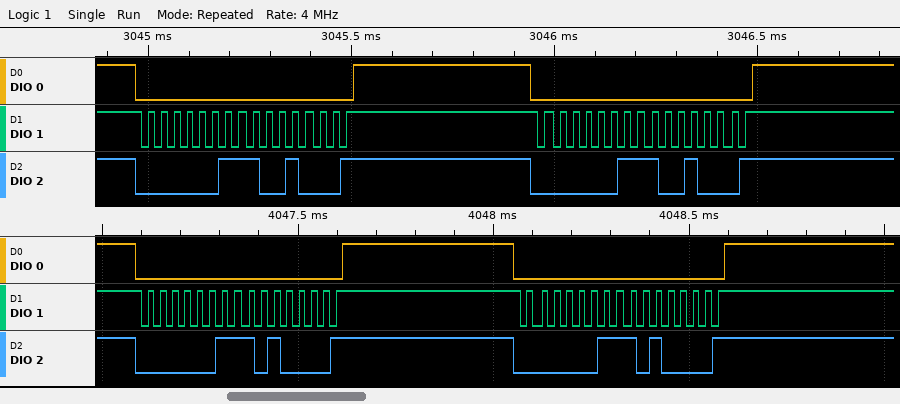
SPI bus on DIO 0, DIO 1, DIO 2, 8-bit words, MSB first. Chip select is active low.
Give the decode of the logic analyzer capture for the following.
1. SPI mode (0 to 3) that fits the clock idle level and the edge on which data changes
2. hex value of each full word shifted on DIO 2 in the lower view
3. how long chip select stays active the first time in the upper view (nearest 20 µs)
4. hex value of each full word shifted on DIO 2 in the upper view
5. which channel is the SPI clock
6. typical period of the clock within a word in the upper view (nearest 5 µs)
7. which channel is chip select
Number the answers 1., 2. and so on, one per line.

1. 3
2. 03, A1, 03, A1
3. 540 µs
4. 03, 91, 03, 91
5. DIO 1
6. 30 µs
7. DIO 0
